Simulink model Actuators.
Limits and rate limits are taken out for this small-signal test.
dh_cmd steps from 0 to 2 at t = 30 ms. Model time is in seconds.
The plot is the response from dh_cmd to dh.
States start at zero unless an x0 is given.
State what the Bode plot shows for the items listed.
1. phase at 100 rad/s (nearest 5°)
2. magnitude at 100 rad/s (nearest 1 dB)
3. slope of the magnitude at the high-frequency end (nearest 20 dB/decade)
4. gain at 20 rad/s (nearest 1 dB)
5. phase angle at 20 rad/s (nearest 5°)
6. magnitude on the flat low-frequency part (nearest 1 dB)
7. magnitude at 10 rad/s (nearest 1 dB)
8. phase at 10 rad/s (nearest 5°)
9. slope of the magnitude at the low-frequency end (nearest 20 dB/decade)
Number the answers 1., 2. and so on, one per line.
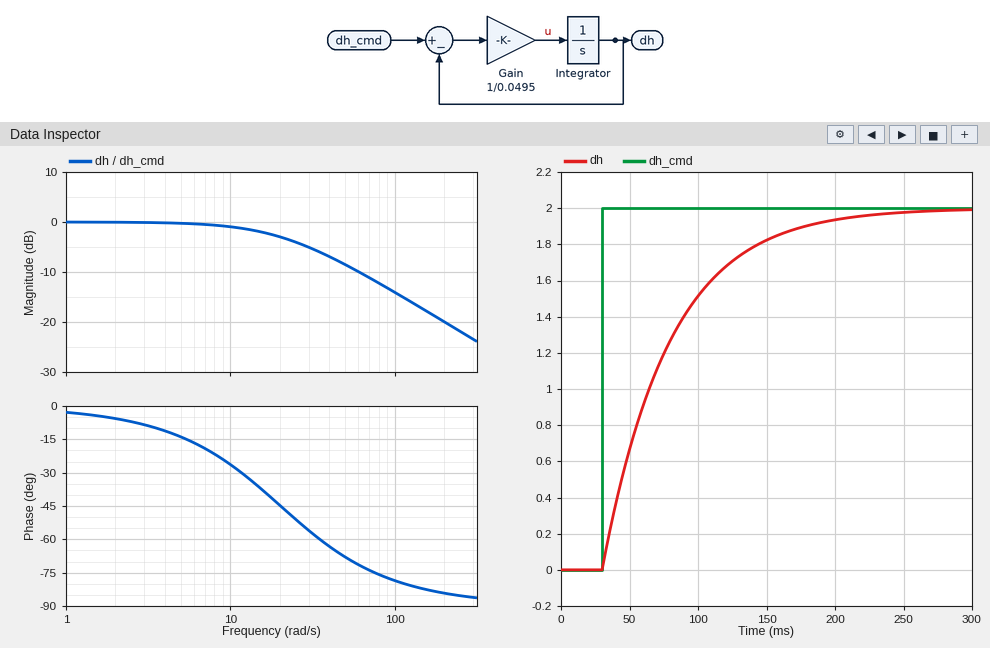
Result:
1. -80°
2. -14 dB
3. -20 dB/decade
4. -3 dB
5. -45°
6. 0 dB
7. -1 dB
8. -25°
9. 0 dB/decade
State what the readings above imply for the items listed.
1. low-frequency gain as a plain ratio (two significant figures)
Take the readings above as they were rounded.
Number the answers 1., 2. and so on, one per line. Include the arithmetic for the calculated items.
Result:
1. 10^(0 / 20) = 1.0
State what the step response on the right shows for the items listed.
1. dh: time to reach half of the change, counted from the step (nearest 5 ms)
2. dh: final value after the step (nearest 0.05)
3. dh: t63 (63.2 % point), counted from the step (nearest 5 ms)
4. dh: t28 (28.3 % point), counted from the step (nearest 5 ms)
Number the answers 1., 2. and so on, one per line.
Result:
1. 35 ms
2. 2.00
3. 50 ms
4. 15 ms
